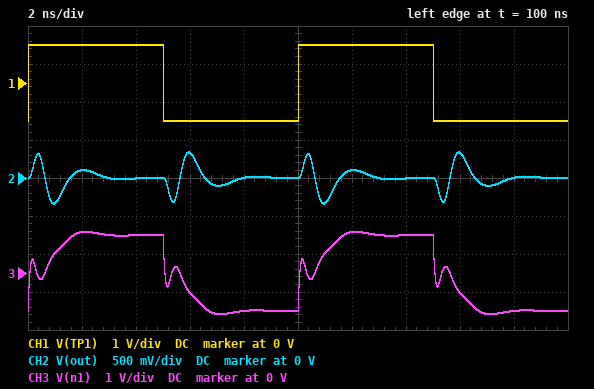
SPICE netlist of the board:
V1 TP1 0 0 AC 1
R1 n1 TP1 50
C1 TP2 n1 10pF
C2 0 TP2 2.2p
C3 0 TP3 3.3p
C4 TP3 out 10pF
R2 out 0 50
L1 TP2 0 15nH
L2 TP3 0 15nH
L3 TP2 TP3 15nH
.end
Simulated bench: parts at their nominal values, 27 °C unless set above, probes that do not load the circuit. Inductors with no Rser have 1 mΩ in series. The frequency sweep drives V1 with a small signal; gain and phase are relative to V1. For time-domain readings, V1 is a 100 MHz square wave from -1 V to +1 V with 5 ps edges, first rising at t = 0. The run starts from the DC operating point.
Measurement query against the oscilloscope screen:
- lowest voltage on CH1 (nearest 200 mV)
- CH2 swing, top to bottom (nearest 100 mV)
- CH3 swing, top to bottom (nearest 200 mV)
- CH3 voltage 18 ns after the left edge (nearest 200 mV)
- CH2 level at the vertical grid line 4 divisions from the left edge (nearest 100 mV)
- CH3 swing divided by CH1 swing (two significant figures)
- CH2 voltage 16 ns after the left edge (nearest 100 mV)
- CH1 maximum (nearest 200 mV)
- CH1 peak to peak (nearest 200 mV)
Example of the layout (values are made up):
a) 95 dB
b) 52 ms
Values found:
a) -1.0 V
b) 700 mV
c) 2.2 V
d) -1.0 V
e) 0 V
f) 1.1
g) 300 mV
h) 1.0 V
i) 2.0 V
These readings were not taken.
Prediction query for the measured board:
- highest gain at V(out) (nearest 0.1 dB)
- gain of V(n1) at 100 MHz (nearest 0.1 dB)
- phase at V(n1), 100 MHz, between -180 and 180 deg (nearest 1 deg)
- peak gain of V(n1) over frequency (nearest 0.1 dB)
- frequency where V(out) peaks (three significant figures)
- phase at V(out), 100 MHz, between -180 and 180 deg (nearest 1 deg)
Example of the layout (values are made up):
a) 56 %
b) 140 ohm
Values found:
a) -6.5 dB
b) -0.4 dB
c) -18 deg
d) 0 dB
e) 694 MHz
f) -126 deg
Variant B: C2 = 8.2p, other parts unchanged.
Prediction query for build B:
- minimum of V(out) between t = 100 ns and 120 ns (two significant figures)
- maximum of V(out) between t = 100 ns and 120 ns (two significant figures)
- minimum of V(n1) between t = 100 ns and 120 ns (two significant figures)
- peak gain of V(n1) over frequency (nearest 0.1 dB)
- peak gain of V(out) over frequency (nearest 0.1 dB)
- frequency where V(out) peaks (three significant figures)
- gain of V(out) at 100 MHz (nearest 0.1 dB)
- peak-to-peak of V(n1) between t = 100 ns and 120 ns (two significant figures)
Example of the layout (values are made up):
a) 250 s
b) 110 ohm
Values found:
a) -310 mV
b) 310 mV
c) -1.2 V
d) 0 dB
e) -6.4 dB
f) 446 MHz
g) -43.9 dB
h) 2.3 V
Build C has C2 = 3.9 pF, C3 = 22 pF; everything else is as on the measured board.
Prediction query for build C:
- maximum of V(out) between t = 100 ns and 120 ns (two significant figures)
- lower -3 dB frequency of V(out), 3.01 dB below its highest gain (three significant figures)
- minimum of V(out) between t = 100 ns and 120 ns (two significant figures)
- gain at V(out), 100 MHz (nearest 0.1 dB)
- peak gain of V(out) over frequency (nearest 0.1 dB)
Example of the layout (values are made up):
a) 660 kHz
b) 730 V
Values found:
a) 240 mV
b) 260 MHz
c) -240 mV
d) -43.4 dB
e) -6.8 dB
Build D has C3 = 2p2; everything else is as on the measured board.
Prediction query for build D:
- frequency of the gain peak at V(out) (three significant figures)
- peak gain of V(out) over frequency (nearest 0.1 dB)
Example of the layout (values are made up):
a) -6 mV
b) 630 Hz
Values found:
a) 753 MHz
b) -6.7 dB
